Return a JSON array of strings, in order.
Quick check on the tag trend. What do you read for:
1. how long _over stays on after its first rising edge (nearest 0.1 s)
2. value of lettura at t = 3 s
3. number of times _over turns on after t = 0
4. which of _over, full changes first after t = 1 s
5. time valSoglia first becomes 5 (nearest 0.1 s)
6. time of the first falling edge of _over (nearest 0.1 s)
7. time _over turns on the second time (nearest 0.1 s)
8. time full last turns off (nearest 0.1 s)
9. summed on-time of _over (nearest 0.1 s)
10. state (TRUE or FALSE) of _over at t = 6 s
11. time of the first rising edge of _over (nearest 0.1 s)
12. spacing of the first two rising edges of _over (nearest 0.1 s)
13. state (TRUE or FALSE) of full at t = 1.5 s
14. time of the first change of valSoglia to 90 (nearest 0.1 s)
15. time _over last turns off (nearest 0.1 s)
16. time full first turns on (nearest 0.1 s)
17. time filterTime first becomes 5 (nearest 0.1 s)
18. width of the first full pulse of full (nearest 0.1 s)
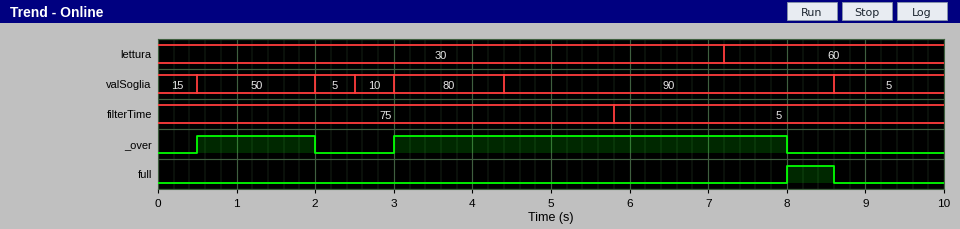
["1.5 s", "30", "2", "_over", "2.0 s", "2.0 s", "3.0 s", "8.6 s", "6.5 s", "TRUE", "0.5 s", "2.5 s", "FALSE", "4.4 s", "8.0 s", "8.0 s", "5.8 s", "0.6 s"]
